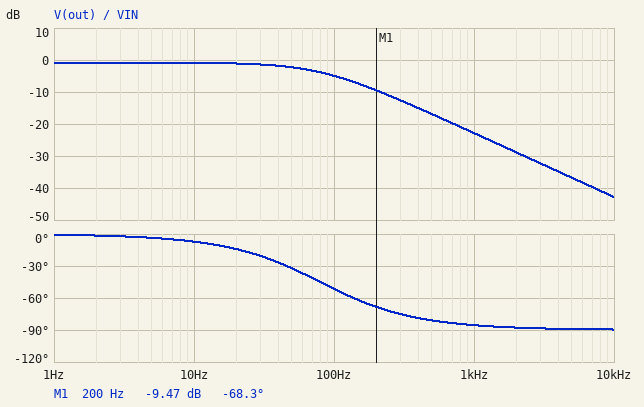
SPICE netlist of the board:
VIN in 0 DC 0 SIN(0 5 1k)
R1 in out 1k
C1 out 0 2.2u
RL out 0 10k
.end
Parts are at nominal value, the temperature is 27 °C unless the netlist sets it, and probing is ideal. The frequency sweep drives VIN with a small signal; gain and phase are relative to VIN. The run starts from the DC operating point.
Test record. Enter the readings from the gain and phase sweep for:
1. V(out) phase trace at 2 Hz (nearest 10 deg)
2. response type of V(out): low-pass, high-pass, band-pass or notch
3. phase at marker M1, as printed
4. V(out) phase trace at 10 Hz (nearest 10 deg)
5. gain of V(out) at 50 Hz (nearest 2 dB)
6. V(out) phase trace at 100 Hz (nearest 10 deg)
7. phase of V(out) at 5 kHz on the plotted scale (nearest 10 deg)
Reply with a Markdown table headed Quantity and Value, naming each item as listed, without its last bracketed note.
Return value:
| Quantity | Value |
|---|---|
| V(out) phase trace at 2 Hz | 0 deg |
| response type of V(out): low-pass, high-pass, band-pass or notch | low-pass |
| phase at marker M1, as printed | -68.3 deg |
| V(out) phase trace at 10 Hz | -10 deg |
| gain of V(out) at 50 Hz | -2 dB |
| V(out) phase trace at 100 Hz | -50 deg |
| phase of V(out) at 5 kHz on the plotted scale | -90 deg |
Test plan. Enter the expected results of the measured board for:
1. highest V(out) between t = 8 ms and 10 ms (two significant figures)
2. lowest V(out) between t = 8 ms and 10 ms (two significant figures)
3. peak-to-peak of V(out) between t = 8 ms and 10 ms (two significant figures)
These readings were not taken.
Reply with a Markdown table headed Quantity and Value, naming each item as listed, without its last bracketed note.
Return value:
| Quantity | Value |
|---|---|
| highest V(out) between t = 8 ms and 10 ms | 370 mV |
| lowest V(out) between t = 8 ms and 10 ms | -360 mV |
| peak-to-peak of V(out) between t = 8 ms and 10 ms | 720 mV |
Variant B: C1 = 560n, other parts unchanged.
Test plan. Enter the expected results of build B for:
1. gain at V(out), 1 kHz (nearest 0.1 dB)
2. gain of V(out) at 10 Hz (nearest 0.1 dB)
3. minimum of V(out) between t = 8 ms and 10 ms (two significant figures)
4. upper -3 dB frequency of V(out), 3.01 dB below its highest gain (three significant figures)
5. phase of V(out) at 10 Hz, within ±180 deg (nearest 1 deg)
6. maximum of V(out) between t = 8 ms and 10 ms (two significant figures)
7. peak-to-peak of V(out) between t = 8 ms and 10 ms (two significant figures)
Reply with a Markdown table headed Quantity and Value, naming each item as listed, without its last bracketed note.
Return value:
| Quantity | Value |
|---|---|
| gain at V(out), 1 kHz | -11.3 dB |
| gain of V(out) at 10 Hz | -0.8 dB |
| minimum of V(out) between t = 8 ms and 10 ms | -1.4 V |
| upper -3 dB frequency of V(out), 3.01 dB below its highest gain | 313 Hz |
| phase of V(out) at 10 Hz, within ±180 deg | -2 deg |
| maximum of V(out) between t = 8 ms and 10 ms | 1.4 V |
| peak-to-peak of V(out) between t = 8 ms and 10 ms | 2.7 V |
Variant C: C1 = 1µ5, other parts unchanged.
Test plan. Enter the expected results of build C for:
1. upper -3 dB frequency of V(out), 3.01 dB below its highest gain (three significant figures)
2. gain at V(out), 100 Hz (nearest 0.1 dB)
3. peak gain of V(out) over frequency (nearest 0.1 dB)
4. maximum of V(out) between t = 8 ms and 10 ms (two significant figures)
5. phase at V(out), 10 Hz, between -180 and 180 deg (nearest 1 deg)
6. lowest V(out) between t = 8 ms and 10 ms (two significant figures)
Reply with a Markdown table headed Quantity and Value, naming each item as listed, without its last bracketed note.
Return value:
| Quantity | Value |
|---|---|
| upper -3 dB frequency of V(out), 3.01 dB below its highest gain | 117 Hz |
| gain at V(out), 100 Hz | -3.2 dB |
| peak gain of V(out) over frequency | -0.8 dB |
| maximum of V(out) between t = 8 ms and 10 ms | 530 mV |
| phase at V(out), 10 Hz, between -180 and 180 deg | -5 deg |
| lowest V(out) between t = 8 ms and 10 ms | -530 mV |
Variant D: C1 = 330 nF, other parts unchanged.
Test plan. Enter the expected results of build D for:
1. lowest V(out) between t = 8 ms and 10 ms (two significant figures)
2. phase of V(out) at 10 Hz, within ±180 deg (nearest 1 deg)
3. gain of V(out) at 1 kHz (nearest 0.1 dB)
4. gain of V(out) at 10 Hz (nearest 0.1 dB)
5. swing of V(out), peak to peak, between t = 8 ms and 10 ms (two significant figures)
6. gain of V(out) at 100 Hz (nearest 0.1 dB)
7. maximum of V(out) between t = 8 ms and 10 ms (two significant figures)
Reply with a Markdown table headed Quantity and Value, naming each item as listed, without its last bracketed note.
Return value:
| Quantity | Value |
|---|---|
| lowest V(out) between t = 8 ms and 10 ms | -2.1 V |
| phase of V(out) at 10 Hz, within ±180 deg | -1 deg |
| gain of V(out) at 1 kHz | -7.4 dB |
| gain of V(out) at 10 Hz | -0.8 dB |
| swing of V(out), peak to peak, between t = 8 ms and 10 ms | 4.3 V |
| gain of V(out) at 100 Hz | -1.0 dB |
| maximum of V(out) between t = 8 ms and 10 ms | 2.1 V |
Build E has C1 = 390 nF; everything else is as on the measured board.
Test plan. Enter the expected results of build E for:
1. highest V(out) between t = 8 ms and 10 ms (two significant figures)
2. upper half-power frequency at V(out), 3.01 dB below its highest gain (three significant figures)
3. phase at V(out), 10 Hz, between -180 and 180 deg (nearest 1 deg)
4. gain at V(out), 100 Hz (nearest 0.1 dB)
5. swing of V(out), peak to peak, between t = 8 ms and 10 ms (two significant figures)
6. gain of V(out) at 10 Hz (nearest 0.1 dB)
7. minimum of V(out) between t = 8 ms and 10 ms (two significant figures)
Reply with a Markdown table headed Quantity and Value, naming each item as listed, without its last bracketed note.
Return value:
| Quantity | Value |
|---|---|
| highest V(out) between t = 8 ms and 10 ms | 1.9 V |
| upper half-power frequency at V(out), 3.01 dB below its highest gain | 449 Hz |
| phase at V(out), 10 Hz, between -180 and 180 deg | -1 deg |
| gain at V(out), 100 Hz | -1.0 dB |
| swing of V(out), peak to peak, between t = 8 ms and 10 ms | 3.7 V |
| gain of V(out) at 10 Hz | -0.8 dB |
| minimum of V(out) between t = 8 ms and 10 ms | -1.9 V |
